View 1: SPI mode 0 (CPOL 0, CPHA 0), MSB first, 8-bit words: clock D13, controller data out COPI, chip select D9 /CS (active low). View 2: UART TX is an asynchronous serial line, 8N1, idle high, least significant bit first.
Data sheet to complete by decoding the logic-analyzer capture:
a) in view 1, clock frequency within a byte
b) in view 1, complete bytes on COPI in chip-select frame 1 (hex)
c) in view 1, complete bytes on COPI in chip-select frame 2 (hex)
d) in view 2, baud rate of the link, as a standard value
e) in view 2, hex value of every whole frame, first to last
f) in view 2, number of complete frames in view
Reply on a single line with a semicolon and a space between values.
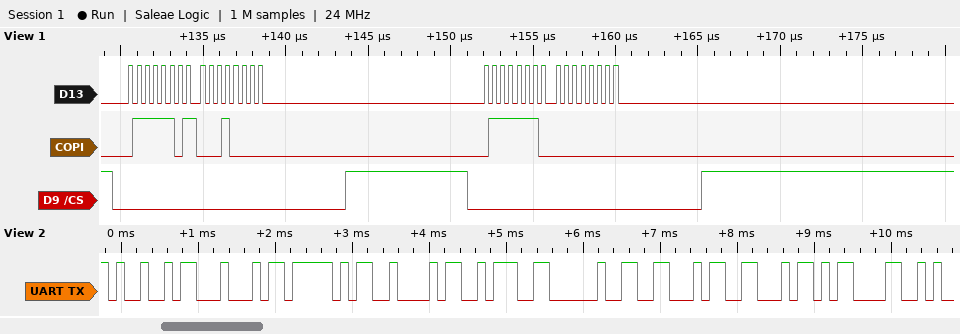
2 MHz; 7D 10; 7E 00; 9600 baud; 0x49 0x44 0x5F 0x42 0x3A 0x20 0x46 0x46 0x0D; 9
